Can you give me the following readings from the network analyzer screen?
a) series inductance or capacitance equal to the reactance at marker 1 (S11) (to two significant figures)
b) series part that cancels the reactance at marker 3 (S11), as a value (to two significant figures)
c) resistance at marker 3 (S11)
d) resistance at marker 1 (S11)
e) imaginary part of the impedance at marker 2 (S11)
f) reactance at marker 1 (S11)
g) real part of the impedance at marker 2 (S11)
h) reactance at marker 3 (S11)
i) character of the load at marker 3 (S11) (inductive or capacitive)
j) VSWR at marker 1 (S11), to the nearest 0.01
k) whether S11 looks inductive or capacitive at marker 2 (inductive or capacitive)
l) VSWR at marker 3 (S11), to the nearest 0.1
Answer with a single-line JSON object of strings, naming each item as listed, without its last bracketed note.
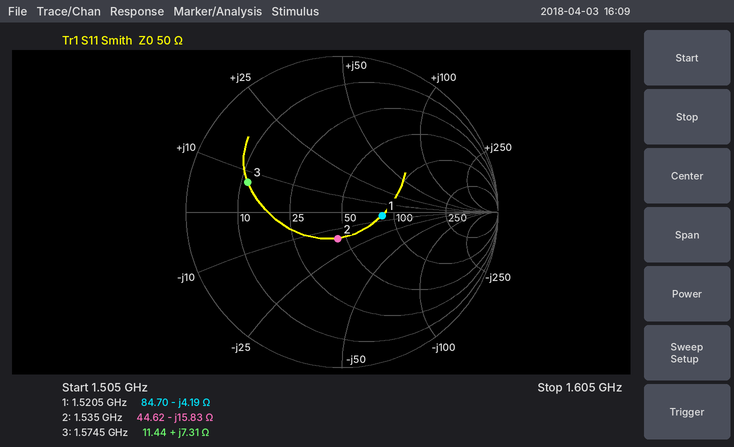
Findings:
{"series inductance or capacitance equal to the reactance at marker 1 (S11)": "25 pF", "series part that cancels the reactance at marker 3 (S11), as a value": "14 pF", "resistance at marker 3": "11.44 Ω", "resistance at marker 1": "84.70 Ω", "imaginary part of the impedance at marker 2": "-15.83 Ω", "reactance at marker 1": "-4.19 Ω", "real part of the impedance at marker 2": "44.62 Ω", "reactance at marker 3": "+7.31 Ω", "character of the load at marker 3 (S11)": "inductive", "VSWR at marker 1 (S11), to the nearest 0.01": "1.70", "whether S11 looks inductive or capacitive at marker 2": "capacitive", "VSWR at marker 3 (S11), to the nearest 0.1": "4.5"}
